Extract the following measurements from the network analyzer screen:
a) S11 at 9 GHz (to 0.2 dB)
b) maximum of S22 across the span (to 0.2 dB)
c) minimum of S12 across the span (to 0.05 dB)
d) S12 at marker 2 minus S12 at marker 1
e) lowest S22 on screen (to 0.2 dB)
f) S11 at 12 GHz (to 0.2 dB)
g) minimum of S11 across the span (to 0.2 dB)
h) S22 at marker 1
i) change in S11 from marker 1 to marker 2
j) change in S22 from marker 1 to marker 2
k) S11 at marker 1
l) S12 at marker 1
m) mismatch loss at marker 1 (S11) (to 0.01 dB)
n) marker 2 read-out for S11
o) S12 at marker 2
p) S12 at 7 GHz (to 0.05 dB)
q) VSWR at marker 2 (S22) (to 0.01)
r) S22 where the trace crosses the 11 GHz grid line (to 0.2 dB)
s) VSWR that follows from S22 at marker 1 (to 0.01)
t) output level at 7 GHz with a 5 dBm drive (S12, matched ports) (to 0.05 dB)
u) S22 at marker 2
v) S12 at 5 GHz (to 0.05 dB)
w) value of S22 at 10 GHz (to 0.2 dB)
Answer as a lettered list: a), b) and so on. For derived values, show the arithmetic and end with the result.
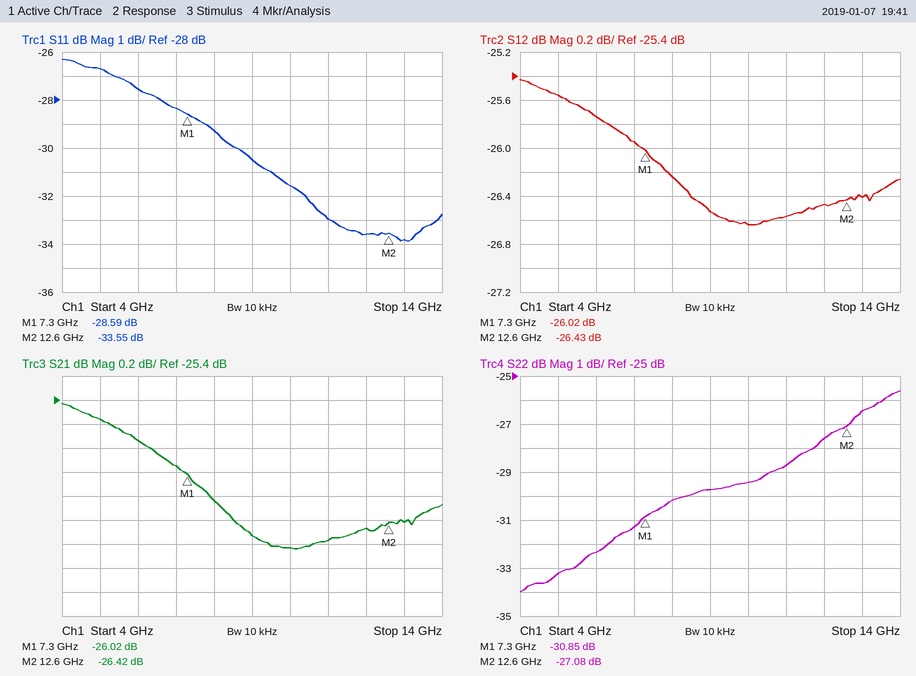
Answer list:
a) -30.4 dB
b) -25.6 dB
c) -26.65 dB
d) -26.43 − (-26.02) = -0.41 dB
e) -34.0 dB
f) -33.6 dB
g) -33.8 dB
h) -30.85 dB
i) -33.55 − (-28.59) = -4.96 dB
j) -27.08 − (-30.85) = 3.77 dB
k) -28.59 dB
l) -26.02 dB
m) −10 log10(1 − 10^(-28.59/10)) ≈ 0.01 dB
n) -33.55 dB
o) -26.43 dB
p) -25.95 dB
q) (1 + 0.0443)/(1 − 0.0443) ≈ 1.09
r) -28.8 dB
s) (1 + 0.0287)/(1 − 0.0287) ≈ 1.06
t) 5 dBm + (-25.95 dB) = -20.95 dBm
u) -27.08 dB
v) -25.55 dB
w) -29.4 dB
